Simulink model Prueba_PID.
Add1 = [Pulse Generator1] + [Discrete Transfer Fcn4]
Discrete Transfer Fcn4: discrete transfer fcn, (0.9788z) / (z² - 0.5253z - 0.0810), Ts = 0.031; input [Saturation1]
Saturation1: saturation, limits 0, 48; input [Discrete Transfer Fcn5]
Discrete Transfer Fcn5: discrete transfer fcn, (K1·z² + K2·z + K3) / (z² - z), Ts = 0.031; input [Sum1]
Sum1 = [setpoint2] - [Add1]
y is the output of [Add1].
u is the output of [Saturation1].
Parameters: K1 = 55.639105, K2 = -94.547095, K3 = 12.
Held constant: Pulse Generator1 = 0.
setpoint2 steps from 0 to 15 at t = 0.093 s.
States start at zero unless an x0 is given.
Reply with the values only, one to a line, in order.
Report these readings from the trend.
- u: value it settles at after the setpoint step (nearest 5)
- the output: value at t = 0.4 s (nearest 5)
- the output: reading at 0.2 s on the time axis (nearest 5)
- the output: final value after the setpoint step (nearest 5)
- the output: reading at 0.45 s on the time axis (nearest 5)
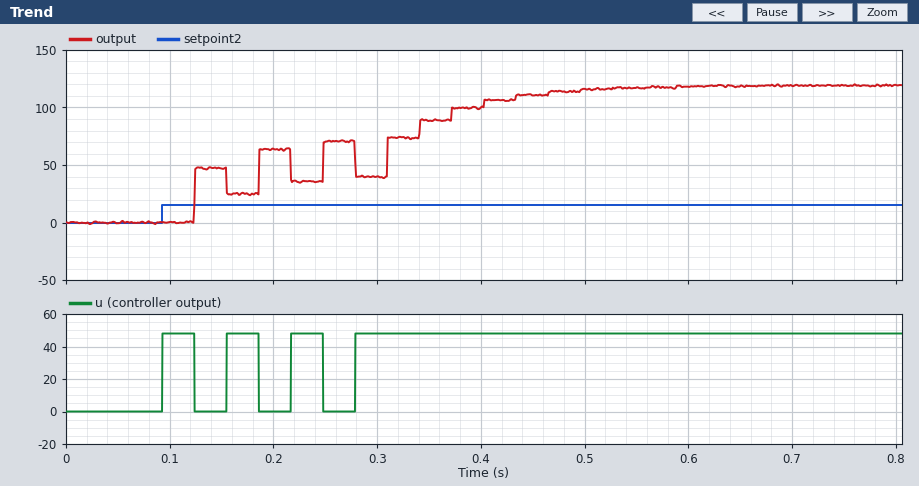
50
100
65
120
110
